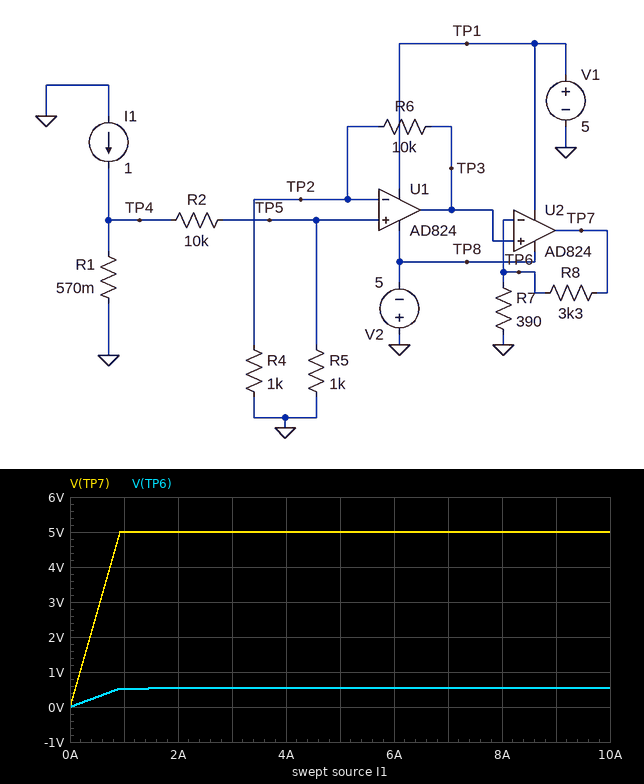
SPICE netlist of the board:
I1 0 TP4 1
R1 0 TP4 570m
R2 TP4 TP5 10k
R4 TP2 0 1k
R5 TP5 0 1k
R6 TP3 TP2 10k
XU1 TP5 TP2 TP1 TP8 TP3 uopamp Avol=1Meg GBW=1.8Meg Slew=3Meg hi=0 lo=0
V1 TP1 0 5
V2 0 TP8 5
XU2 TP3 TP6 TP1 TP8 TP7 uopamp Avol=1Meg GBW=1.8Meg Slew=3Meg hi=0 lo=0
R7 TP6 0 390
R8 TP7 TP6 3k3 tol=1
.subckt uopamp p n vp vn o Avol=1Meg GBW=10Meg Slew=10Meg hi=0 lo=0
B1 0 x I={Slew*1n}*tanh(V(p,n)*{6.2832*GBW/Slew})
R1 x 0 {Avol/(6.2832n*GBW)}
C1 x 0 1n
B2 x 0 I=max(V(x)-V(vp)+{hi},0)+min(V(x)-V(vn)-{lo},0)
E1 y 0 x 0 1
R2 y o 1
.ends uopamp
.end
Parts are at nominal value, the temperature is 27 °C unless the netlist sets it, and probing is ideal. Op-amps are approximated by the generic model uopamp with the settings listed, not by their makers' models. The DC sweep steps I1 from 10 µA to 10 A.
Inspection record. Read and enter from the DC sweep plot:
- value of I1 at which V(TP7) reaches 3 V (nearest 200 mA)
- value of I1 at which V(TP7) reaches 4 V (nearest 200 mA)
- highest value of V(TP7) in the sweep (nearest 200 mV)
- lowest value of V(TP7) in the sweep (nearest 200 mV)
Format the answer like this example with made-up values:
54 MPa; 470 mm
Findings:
600 mA; 800 mA; 5.0 V; 0 V
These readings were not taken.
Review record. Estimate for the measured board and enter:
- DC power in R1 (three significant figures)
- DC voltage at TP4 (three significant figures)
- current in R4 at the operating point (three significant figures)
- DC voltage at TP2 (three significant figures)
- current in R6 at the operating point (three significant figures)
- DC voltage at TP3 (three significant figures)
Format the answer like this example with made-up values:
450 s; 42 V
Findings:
570 mW; 570 mV; 51.8 µA; 51.8 mV; 51.8 µA; 570 mV
